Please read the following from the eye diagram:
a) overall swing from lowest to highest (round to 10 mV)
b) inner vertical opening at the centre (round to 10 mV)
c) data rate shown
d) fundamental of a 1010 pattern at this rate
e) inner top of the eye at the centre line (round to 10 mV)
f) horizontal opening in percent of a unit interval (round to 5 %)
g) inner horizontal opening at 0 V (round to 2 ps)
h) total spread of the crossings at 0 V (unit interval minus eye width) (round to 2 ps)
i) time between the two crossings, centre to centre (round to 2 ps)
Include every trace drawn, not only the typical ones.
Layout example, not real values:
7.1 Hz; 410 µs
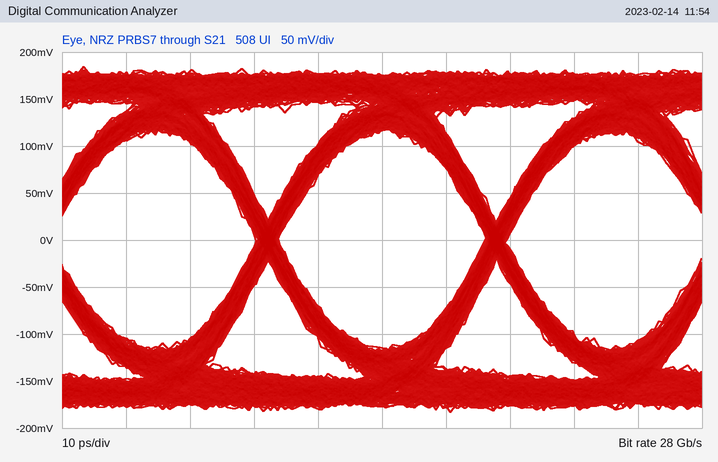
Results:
370 mV; 230 mV; 28 Gb/s; 14 GHz; 120 mV; 90 %; 32 ps; 4 ps; 36 ps
